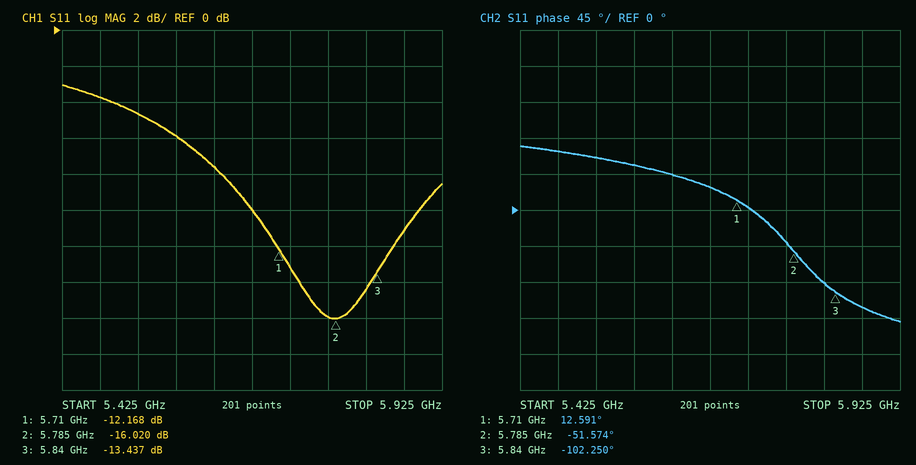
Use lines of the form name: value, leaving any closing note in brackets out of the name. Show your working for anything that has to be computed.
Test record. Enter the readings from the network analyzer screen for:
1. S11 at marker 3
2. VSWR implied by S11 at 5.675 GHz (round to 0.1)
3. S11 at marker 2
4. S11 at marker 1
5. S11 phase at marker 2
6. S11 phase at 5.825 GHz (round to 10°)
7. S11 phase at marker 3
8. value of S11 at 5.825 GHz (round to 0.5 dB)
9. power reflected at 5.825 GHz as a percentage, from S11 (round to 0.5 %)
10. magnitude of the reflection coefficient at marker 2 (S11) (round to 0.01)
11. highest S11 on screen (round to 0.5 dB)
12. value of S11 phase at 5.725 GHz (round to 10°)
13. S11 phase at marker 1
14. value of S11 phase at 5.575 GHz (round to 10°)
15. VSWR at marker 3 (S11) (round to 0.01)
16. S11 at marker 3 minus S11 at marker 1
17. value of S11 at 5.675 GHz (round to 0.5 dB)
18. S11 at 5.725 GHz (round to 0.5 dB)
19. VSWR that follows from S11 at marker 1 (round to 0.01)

S11 at marker 3: -13.437 dB
VSWR implied by S11 at 5.675 GHz: |Γ| = 10^(-10/20) = 0.3162; VSWR = (1 + 0.3162)/(1 − 0.3162) ≈ 1.9
S11 at marker 2: -16.020 dB
S11 at marker 1: -12.168 dB
S11 phase at marker 2: -51.574°
S11 phase at 5.825 GHz: -90°
S11 phase at marker 3: -102.250°
value of S11 at 5.825 GHz: -14.5 dB
power reflected at 5.825 GHz as a percentage, from S11: 10^(-14.5/10) ≈ 3.5 %
magnitude of the reflection coefficient at marker 2 (S11): 10^(-16.02/20) ≈ 0.16
highest S11 on screen: -3.0 dB
value of S11 phase at 5.725 GHz: 0°
S11 phase at marker 1: 12.591°
value of S11 phase at 5.575 GHz: 60°
VSWR at marker 3 (S11): (1 + 0.2129)/(1 − 0.2129) ≈ 1.54
S11 at marker 3 minus S11 at marker 1: -13.437 − (-12.168) = -1.269 dB
value of S11 at 5.675 GHz: -10.0 dB
S11 at 5.725 GHz: -13.0 dB
VSWR that follows from S11 at marker 1: (1 + 0.2464)/(1 − 0.2464) ≈ 1.65
